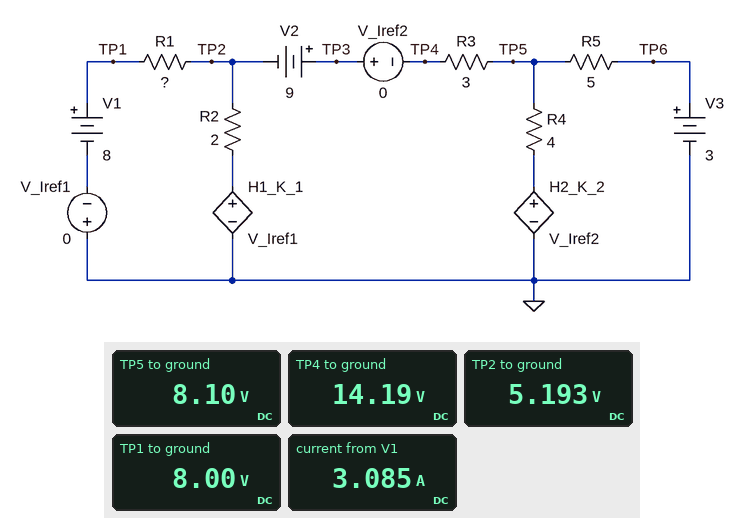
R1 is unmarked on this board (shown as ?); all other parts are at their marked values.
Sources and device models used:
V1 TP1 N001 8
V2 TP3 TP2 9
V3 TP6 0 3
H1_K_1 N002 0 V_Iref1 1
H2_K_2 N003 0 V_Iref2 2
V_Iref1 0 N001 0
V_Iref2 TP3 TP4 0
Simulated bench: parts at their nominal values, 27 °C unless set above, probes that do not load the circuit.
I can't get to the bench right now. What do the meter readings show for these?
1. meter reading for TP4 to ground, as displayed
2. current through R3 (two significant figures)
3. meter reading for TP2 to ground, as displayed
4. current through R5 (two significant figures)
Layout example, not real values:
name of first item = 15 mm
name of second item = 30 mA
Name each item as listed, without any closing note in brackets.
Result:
meter reading for TP4 to ground, as displayed = 14.19 V
current through R3 = 2.0 A
meter reading for TP2 to ground, as displayed = 5.193 V
current through R5 = 1.0 A
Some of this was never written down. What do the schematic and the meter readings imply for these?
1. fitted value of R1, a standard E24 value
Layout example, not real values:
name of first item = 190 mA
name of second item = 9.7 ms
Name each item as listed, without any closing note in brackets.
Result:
fitted value of R1, a standard E24 value = 0.91 Ω
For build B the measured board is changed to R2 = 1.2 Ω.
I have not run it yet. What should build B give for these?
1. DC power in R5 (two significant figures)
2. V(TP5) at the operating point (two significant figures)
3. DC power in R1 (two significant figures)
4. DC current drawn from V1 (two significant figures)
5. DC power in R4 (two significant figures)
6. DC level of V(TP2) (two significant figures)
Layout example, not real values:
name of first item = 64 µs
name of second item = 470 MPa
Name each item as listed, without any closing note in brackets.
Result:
DC power in R5 = 5.0 W
V(TP5) at the operating point = 8.0 V
DC power in R1 = 10 W
DC current drawn from V1 = 3.3 A
DC power in R4 = 4.0 W
DC level of V(TP2) = 5.0 V
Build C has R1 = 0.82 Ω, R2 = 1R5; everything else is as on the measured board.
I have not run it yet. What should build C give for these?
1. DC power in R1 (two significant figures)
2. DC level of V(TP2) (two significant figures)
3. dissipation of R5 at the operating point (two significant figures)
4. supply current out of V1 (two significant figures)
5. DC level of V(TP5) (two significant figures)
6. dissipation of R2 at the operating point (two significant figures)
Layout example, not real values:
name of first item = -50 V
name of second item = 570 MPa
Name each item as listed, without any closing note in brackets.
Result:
DC power in R1 = 9.1 W
DC level of V(TP2) = 5.3 V
dissipation of R5 at the operating point = 5.3 W
supply current out of V1 = 3.3 A
DC level of V(TP5) = 8.1 V
dissipation of R2 at the operating point = 2.5 W
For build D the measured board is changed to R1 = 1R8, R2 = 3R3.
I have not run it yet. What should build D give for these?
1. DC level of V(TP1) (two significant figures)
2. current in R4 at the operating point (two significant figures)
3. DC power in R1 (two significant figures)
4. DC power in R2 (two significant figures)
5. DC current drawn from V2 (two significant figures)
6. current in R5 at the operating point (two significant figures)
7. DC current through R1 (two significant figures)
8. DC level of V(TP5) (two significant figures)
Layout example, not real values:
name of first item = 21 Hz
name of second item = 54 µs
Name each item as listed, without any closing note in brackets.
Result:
DC level of V(TP1) = 8.0 V
current in R4 at the operating point = 940 mA
DC power in R1 = 9.5 W
DC power in R2 = 750 mW
DC current drawn from V2 = 1.8 A
current in R5 at the operating point = 880 mA
DC current through R1 = 2.3 A
DC level of V(TP5) = 7.4 V
